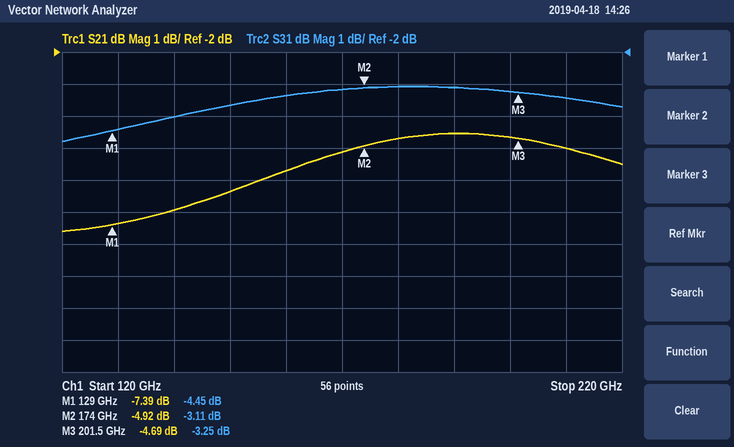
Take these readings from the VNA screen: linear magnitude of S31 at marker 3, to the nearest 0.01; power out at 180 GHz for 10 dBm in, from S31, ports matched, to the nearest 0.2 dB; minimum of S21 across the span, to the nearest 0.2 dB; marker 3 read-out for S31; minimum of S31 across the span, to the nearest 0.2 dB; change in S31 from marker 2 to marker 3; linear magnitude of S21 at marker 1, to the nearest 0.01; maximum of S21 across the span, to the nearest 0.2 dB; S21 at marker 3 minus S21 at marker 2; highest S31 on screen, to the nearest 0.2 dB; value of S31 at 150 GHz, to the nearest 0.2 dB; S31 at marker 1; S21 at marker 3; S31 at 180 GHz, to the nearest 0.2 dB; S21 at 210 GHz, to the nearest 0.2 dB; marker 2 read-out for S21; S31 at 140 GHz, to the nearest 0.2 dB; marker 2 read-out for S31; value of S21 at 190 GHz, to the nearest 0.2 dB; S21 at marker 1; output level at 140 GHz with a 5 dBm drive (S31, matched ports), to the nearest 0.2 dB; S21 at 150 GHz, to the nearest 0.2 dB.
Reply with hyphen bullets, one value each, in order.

- 0.69
- 7.0 dBm
- -7.6 dB
- -3.25 dB
- -4.8 dB
- -0.14 dB
- 0.43
- -4.6 dB
- 0.23 dB
- -3.0 dB
- -3.6 dB
- -4.45 dB
- -4.69 dB
- -3.0 dB
- -5.0 dB
- -4.92 dB
- -4.0 dB
- -3.11 dB
- -4.6 dB
- -7.39 dB
- 1.0 dBm
- -6.4 dB
